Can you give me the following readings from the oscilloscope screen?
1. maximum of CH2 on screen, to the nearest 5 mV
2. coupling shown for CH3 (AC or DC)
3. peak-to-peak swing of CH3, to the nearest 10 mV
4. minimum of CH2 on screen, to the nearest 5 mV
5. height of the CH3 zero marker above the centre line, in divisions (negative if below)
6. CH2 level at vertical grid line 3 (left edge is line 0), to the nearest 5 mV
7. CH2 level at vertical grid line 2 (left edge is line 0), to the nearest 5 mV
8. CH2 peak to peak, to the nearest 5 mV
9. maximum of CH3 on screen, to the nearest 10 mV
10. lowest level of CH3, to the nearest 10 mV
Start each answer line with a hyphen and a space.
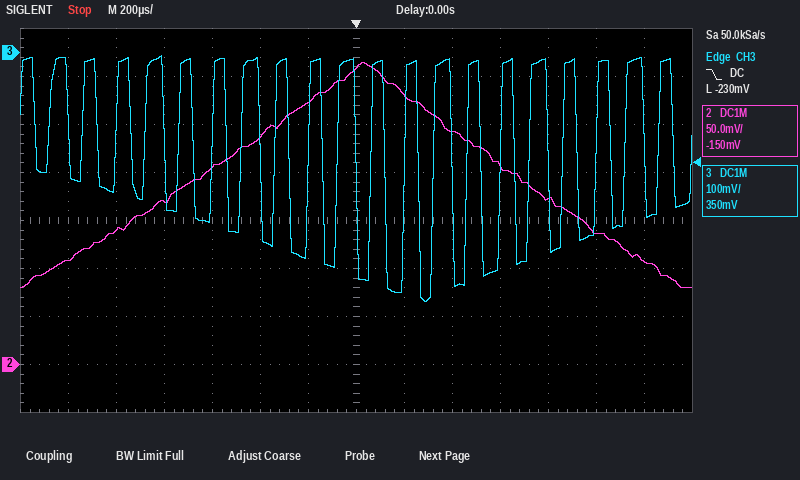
- 315 mV
- DC
- 510 mV
- 80 mV
- +3.5 div
- 170 mV
- 140 mV
- 235 mV
- -10 mV
- -520 mV
